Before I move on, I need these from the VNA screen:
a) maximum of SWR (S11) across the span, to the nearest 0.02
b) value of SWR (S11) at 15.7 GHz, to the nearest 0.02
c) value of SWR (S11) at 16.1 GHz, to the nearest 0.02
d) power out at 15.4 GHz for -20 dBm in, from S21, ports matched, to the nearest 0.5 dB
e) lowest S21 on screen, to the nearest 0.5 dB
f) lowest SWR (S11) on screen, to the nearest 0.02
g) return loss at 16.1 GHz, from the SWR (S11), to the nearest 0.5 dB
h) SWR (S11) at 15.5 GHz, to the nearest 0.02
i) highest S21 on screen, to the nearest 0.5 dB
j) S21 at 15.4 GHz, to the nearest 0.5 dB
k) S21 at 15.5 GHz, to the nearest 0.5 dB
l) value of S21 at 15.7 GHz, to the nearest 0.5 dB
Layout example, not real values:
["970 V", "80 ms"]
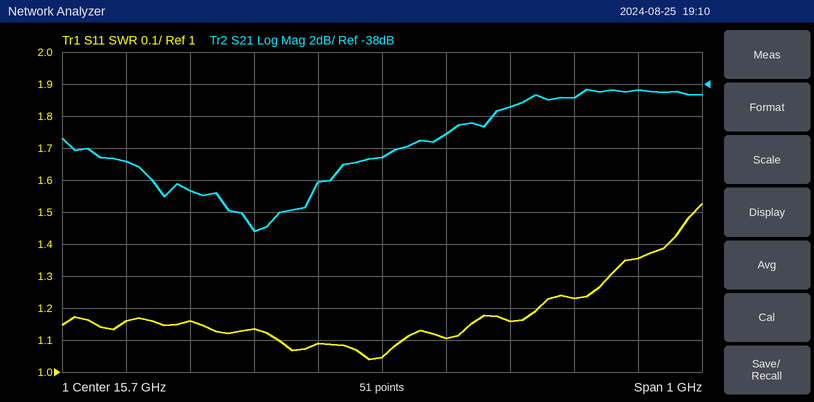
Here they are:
["1.52", "1.04", "1.36", "-64.5 dBm", "-47.0 dB", "1.04", "16.5 dB", "1.14", "-38.5 dB", "-44.5 dB", "-47.0 dB", "-42.5 dB"]
